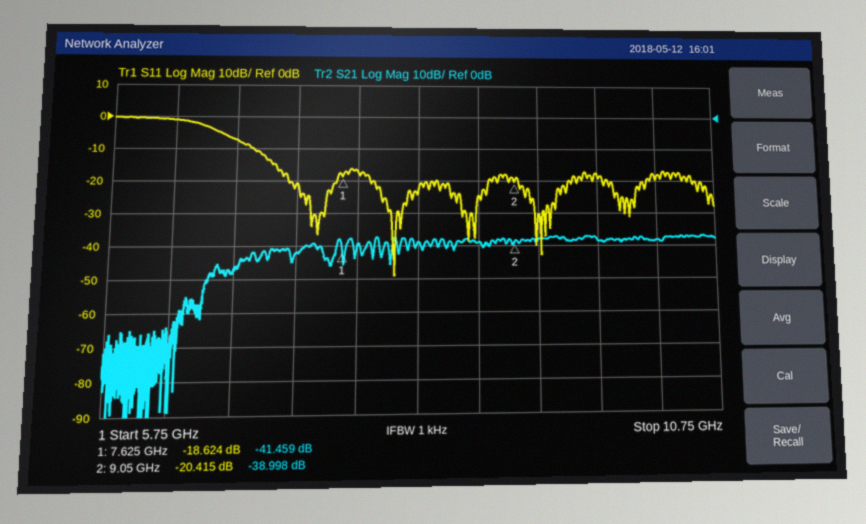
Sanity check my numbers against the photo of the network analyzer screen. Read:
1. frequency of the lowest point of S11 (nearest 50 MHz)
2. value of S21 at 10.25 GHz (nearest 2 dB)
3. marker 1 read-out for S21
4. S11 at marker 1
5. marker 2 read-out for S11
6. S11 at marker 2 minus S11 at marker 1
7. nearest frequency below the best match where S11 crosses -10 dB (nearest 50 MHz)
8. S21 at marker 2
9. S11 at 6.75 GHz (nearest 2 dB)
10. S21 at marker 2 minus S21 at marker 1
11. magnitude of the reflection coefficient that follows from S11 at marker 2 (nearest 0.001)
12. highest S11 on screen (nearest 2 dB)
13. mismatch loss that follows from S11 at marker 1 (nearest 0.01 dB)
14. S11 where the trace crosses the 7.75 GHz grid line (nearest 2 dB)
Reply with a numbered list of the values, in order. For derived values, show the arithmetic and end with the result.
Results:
1. 8.05 GHz
2. -38 dB
3. -41.459 dB
4. -18.624 dB
5. -20.415 dB
6. -20.415 − (-18.624) = -1.791 dB
7. 6.90 GHz
8. -38.998 dB
9. -8 dB
10. -38.998 − (-41.459) = 2.461 dB
11. 10^(-20.415/20) ≈ 0.095
12. 0 dB
13. −10 log10(1 − 10^(-18.624/10)) ≈ 0.06 dB
14. -18 dB
